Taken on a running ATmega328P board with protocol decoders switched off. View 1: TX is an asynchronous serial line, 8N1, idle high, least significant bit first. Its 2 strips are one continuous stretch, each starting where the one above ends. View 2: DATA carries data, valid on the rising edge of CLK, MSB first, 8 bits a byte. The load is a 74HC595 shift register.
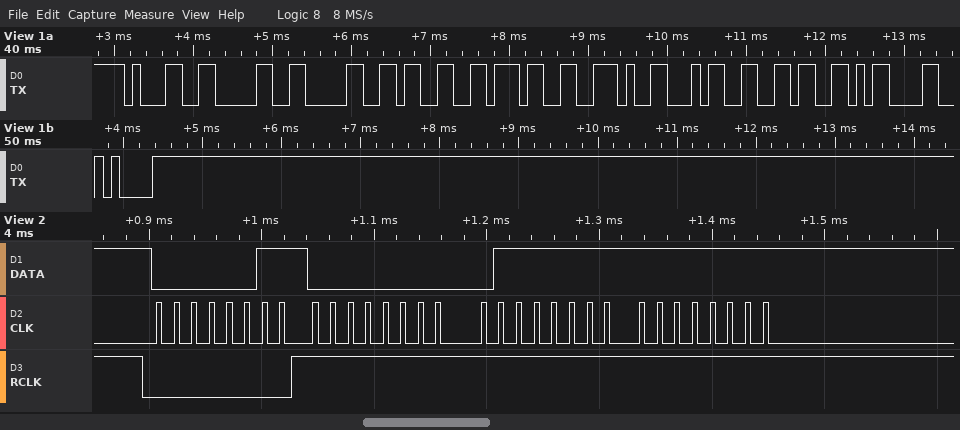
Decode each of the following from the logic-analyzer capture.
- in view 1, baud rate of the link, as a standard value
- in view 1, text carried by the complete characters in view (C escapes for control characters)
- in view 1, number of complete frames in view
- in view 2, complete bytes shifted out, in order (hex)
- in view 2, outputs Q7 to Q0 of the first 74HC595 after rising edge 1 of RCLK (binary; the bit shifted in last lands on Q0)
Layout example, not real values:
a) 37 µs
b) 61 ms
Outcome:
a) 9600 baud
b) "10037.46\r\n"
c) 10
d) 0x03 0x00 0x7F 0xFF
e) 00000011
